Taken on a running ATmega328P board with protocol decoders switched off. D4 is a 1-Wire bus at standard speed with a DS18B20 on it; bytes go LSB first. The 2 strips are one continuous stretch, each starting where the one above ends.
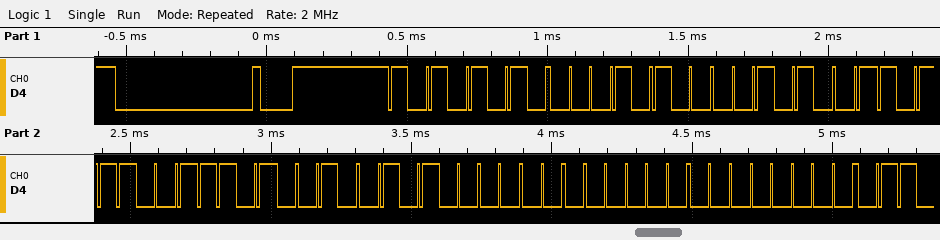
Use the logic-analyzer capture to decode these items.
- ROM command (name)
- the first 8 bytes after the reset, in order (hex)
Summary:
Match ROM
55 28 94 9D 4B 0A 00 00
